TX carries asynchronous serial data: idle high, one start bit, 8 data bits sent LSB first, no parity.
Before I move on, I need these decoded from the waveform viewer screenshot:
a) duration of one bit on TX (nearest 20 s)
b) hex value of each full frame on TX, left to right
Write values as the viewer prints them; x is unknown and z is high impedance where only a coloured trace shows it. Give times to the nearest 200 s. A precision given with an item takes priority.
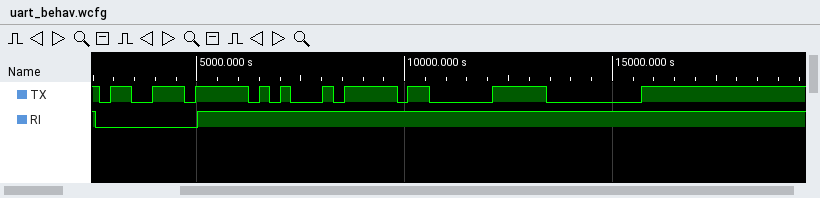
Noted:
260 s
73, 45, 03, 00
